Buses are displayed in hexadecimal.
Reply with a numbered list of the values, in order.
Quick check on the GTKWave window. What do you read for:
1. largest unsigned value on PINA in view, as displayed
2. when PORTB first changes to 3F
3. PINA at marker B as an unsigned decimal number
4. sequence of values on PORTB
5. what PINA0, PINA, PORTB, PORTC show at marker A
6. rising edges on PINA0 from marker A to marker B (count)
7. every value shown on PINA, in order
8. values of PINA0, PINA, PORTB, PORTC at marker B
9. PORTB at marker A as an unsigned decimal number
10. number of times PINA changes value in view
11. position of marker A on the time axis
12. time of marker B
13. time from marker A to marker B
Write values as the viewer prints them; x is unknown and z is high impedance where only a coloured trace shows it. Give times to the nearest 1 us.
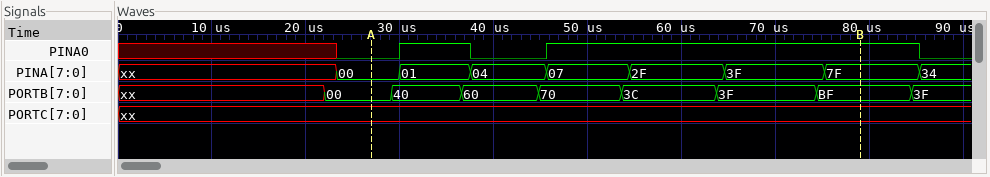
1. 7F
2. 64 us
3. 127
4. xx, 00, 40, 60, 70, 3C, 3F, BF, 3F
5. PINA0=0, PINA=00, PORTB=00, PORTC=xx
6. 2
7. xx, 00, 01, 04, 07, 2F, 3F, 7F, 34
8. PINA0=1, PINA=7F, PORTB=BF, PORTC=xx
9. 0
10. 8
11. 27 us
12. 79 us
13. 52 us
